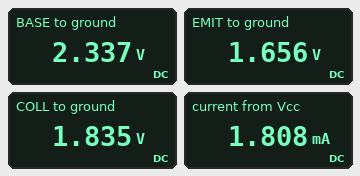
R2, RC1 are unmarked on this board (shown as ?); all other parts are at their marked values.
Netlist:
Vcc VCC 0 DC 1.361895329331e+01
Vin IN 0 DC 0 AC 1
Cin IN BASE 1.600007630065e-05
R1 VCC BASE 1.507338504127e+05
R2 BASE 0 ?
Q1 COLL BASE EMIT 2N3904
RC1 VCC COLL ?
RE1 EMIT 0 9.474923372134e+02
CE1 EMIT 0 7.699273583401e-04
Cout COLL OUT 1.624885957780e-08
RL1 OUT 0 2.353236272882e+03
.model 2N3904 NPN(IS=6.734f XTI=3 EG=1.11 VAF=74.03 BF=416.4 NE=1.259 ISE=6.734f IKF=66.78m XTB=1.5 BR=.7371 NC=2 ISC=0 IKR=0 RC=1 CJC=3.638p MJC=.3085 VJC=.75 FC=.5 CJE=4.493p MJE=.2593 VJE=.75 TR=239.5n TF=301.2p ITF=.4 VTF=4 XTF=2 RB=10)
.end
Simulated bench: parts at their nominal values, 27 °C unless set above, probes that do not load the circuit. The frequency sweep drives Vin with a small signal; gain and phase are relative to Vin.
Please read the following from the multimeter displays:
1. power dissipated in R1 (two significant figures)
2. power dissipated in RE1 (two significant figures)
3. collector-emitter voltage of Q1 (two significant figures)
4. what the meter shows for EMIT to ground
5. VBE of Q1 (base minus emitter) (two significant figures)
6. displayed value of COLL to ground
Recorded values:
840 µW
2.9 mW
180 mV
1.656 V
680 mV
1.835 V
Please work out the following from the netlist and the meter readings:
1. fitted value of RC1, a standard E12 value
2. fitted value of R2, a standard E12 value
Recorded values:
6.8 kΩ
39 kΩ
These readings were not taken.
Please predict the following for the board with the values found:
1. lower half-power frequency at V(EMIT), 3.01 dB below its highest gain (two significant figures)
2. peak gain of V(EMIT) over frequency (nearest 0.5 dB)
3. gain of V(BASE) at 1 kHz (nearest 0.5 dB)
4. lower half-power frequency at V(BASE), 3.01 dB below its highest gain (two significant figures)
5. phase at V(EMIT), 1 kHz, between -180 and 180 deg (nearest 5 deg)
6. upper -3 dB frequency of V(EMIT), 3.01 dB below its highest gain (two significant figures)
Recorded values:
250 mHz
-26.5 dB
0 dB
170 Hz
-75 deg
180 Hz
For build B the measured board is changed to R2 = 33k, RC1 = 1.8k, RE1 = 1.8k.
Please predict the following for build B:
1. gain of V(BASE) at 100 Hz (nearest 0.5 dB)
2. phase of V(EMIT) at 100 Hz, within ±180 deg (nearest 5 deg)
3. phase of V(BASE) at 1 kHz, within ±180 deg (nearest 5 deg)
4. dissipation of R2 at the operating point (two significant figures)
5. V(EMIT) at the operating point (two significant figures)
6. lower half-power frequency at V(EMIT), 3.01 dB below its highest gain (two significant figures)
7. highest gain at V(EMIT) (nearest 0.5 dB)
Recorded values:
0 dB
-85 deg
0 deg
160 µW
1.6 V
290 mHz
-2.5 dB
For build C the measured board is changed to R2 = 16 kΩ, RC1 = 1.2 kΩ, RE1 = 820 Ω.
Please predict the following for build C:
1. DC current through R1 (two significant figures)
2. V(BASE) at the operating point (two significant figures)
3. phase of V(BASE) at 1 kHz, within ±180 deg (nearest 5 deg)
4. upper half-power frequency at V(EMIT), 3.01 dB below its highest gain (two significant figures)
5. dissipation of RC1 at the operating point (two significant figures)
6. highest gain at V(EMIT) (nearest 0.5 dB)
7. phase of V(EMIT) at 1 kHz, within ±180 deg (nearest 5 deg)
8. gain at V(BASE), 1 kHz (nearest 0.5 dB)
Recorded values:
82 µA
1.2 V
0 deg
8.6 Hz
600 µW
-3.5 dB
-90 deg
0 dB
